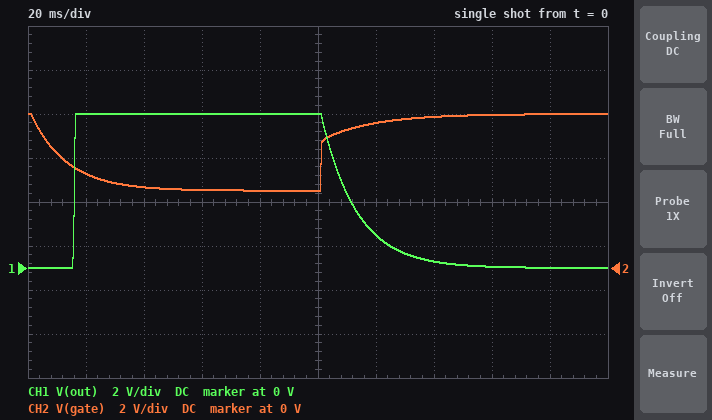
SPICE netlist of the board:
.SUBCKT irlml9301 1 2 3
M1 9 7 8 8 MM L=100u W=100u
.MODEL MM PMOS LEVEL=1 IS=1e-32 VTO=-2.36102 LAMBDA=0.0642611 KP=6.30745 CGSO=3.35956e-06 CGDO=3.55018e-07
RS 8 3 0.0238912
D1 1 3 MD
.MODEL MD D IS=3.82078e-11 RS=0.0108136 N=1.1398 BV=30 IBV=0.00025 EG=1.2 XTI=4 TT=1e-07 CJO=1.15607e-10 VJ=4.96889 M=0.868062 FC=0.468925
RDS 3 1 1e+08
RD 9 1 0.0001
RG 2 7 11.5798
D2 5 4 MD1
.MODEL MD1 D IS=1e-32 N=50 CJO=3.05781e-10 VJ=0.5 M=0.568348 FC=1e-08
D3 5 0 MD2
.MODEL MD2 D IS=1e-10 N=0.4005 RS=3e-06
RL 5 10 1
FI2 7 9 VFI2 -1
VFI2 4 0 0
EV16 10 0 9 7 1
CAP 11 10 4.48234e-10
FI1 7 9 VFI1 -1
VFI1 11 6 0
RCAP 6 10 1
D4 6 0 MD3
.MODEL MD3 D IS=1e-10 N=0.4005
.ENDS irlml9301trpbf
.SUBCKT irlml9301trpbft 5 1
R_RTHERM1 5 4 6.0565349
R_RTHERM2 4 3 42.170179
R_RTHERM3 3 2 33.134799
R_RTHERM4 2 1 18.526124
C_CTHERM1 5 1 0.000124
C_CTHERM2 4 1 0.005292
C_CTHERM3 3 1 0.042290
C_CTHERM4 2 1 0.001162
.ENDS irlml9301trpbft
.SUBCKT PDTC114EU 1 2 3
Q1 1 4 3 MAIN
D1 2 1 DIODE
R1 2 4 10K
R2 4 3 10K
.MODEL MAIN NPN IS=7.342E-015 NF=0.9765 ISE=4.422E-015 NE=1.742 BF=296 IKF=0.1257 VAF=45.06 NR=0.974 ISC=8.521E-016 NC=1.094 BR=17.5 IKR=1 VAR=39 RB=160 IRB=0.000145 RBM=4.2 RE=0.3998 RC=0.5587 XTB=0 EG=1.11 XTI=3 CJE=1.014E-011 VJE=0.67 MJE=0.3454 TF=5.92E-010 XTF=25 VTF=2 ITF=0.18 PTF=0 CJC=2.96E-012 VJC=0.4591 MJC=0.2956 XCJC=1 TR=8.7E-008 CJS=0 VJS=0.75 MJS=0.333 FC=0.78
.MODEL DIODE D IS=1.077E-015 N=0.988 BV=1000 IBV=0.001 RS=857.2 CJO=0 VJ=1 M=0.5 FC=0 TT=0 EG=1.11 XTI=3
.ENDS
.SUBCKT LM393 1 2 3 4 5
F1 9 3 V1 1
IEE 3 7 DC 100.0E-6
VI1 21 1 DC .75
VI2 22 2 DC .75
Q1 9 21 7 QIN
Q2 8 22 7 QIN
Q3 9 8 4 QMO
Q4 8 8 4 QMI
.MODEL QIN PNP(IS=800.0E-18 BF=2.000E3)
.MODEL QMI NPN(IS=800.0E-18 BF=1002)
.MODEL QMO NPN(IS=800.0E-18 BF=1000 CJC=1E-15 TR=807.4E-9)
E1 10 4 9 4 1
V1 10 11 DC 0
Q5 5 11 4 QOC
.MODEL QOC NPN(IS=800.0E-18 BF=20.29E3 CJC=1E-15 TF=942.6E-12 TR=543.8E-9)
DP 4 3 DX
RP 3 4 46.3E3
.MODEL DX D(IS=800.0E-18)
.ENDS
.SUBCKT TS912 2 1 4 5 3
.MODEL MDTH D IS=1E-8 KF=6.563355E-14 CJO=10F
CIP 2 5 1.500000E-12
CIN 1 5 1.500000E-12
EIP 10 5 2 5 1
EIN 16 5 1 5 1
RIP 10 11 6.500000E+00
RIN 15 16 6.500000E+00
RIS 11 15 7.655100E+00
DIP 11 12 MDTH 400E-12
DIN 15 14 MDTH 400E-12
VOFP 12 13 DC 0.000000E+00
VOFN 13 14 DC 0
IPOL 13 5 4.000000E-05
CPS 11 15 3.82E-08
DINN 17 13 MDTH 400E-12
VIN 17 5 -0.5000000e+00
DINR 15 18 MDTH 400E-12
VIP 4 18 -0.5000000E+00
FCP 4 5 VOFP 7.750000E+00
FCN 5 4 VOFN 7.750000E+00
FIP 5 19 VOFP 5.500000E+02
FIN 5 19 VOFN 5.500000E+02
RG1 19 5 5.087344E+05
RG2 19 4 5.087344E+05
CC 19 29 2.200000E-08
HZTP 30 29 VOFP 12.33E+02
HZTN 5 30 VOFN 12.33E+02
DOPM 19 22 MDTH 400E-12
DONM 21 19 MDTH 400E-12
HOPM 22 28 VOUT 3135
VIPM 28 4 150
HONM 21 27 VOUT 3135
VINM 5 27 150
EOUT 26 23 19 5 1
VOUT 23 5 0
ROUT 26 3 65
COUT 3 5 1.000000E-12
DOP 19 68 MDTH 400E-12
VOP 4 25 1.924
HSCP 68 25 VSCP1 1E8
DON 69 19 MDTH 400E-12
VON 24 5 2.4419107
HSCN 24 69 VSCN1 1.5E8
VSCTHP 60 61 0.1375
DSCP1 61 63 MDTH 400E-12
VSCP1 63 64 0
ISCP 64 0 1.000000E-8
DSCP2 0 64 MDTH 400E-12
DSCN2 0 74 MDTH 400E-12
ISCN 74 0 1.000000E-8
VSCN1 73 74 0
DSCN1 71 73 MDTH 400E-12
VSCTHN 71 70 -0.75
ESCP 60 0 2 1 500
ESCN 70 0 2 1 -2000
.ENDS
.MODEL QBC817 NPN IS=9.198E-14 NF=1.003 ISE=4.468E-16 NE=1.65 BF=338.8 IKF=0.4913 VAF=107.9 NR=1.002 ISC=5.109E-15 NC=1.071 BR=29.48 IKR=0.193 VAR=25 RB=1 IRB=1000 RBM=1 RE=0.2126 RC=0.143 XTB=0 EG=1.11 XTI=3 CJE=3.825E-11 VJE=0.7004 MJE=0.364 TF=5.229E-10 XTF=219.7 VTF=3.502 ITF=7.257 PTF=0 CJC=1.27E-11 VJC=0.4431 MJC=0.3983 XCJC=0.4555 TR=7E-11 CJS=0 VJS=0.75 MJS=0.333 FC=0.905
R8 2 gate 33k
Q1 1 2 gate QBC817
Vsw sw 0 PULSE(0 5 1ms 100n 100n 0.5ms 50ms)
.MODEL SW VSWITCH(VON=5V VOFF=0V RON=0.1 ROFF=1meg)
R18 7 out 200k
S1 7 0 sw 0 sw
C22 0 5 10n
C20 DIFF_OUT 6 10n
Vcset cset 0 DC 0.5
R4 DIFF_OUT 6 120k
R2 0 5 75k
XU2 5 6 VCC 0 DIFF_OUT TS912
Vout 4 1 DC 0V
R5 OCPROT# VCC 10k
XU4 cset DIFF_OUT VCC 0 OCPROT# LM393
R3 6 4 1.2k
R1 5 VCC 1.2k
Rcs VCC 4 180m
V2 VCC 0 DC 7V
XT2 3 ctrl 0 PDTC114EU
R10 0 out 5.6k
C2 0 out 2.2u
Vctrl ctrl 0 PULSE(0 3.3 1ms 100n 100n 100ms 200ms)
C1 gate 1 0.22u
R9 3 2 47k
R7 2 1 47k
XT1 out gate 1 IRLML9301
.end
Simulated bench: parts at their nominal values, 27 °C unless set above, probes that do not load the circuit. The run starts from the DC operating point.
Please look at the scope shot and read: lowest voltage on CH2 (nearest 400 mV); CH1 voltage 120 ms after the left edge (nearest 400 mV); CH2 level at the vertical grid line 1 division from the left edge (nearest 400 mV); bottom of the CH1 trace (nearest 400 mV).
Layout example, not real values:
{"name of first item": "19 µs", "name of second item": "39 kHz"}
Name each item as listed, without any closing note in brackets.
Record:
{"lowest voltage on CH2": "3.6 V", "CH1 voltage 120 ms after the left edge": "1.6 V", "CH2 level at the vertical grid line 1 division from the left edge": "4.4 V", "bottom of the CH1 trace": "0 V"}
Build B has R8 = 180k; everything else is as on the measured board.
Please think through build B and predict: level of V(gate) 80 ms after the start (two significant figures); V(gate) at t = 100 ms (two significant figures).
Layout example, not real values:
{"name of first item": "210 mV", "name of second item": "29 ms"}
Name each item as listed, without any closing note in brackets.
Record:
{"level of V(gate) 80 ms after the start": "4.1 V", "V(gate) at t = 100 ms": "3.9 V"}
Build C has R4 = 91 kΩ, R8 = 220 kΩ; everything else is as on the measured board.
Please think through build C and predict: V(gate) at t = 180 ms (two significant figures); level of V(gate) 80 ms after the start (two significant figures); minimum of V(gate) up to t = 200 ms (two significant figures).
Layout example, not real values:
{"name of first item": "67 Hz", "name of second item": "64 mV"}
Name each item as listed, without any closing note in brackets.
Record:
{"V(gate) at t = 180 ms": "6.9 V", "level of V(gate) 80 ms after the start": "4.3 V", "minimum of V(gate) up to t = 200 ms": "4.1 V"}
